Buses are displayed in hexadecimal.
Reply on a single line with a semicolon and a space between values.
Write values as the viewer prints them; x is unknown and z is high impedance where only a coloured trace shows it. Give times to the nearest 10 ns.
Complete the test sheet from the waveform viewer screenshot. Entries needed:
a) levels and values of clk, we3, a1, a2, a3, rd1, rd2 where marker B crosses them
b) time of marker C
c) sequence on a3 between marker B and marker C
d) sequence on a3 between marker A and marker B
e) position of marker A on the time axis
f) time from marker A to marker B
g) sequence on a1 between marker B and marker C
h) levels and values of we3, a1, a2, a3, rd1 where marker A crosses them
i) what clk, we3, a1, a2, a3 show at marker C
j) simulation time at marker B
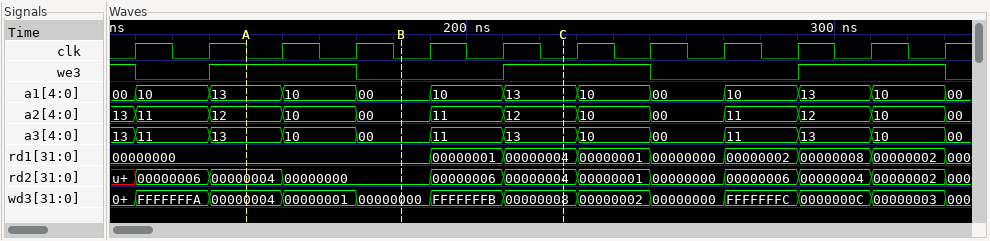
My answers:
clk=0, we3=0, a1=00, a2=00, a3=00, rd1=00000000, rd2=00000000; 230 ns; 00, 11, 13; 13, 10, 00; 140 ns; 40 ns; 00, 10, 13; we3=1, a1=13, a2=12, a3=13, rd1=00000000; clk=0, we3=1, a1=13, a2=12, a3=13; 180 ns
